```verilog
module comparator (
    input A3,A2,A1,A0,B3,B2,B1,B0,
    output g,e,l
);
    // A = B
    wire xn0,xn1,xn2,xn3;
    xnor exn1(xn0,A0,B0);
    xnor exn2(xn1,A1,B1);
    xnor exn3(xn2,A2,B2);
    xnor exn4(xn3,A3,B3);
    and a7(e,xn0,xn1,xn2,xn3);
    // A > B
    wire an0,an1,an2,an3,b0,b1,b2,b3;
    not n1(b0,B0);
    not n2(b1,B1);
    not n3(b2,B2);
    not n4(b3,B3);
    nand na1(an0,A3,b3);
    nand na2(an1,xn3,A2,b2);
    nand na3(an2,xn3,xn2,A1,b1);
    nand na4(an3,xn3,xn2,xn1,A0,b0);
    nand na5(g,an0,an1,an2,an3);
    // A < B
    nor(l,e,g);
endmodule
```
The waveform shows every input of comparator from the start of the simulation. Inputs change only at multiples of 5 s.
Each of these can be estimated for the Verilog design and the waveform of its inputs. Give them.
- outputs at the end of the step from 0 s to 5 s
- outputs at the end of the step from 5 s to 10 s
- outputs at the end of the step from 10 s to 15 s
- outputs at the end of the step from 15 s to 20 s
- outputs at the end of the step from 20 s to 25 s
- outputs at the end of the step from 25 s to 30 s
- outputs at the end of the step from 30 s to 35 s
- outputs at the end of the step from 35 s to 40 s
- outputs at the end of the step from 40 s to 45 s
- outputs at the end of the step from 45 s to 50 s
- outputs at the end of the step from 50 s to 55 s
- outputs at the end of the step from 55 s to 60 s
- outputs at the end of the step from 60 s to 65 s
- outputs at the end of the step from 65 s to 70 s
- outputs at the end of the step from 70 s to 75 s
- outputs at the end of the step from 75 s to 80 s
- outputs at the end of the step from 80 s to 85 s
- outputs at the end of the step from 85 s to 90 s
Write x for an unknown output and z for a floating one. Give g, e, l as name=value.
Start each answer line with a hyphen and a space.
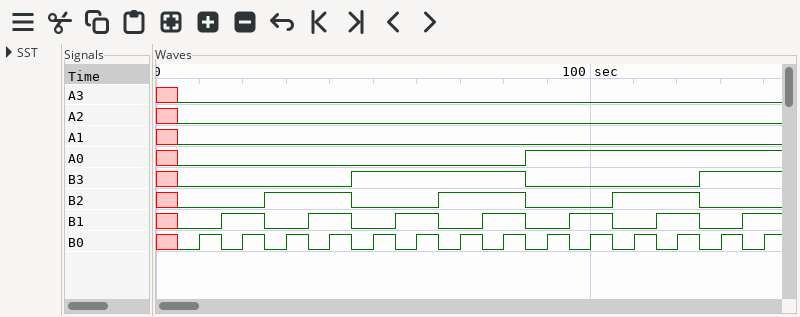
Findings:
- g=x, e=x, l=x
- g=0, e=1, l=0
- g=0, e=0, l=1
- g=0, e=0, l=1
- g=0, e=0, l=1
- g=0, e=0, l=1
- g=0, e=0, l=1
- g=0, e=0, l=1
- g=0, e=0, l=1
- g=0, e=0, l=1
- g=0, e=0, l=1
- g=0, e=0, l=1
- g=0, e=0, l=1
- g=0, e=0, l=1
- g=0, e=0, l=1
- g=0, e=0, l=1
- g=0, e=0, l=1
- g=1, e=0, l=0
